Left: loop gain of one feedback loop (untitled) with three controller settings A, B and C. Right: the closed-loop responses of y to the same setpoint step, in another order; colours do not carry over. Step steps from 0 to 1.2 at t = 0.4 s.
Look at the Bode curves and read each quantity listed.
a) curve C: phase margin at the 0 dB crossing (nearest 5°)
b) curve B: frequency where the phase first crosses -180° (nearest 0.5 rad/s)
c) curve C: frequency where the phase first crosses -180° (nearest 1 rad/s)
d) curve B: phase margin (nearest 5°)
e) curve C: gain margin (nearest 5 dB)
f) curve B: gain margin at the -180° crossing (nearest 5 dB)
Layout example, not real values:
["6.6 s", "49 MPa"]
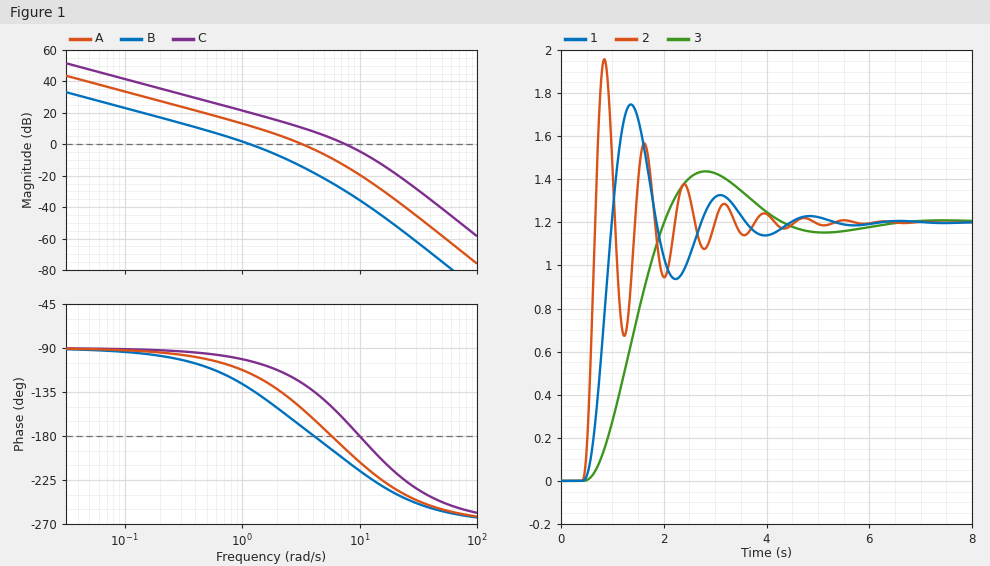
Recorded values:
["15°", "4.0 rad/s", "10 rad/s", "50°", "5 dB", "20 dB"]
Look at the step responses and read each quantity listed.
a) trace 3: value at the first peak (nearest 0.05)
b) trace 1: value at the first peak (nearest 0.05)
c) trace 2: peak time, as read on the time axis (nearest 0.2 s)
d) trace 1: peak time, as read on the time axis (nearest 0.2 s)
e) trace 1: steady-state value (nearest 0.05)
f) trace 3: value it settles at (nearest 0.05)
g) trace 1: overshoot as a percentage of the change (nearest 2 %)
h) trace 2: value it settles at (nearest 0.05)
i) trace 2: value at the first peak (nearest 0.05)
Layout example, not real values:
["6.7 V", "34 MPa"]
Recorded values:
["1.45", "1.75", "0.8 s", "1.4 s", "1.20", "1.20", "46 %", "1.20", "1.95"]
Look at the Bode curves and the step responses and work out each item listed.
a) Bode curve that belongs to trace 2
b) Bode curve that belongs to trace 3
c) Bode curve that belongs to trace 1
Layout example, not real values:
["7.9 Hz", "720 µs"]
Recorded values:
["C", "B", "A"]
